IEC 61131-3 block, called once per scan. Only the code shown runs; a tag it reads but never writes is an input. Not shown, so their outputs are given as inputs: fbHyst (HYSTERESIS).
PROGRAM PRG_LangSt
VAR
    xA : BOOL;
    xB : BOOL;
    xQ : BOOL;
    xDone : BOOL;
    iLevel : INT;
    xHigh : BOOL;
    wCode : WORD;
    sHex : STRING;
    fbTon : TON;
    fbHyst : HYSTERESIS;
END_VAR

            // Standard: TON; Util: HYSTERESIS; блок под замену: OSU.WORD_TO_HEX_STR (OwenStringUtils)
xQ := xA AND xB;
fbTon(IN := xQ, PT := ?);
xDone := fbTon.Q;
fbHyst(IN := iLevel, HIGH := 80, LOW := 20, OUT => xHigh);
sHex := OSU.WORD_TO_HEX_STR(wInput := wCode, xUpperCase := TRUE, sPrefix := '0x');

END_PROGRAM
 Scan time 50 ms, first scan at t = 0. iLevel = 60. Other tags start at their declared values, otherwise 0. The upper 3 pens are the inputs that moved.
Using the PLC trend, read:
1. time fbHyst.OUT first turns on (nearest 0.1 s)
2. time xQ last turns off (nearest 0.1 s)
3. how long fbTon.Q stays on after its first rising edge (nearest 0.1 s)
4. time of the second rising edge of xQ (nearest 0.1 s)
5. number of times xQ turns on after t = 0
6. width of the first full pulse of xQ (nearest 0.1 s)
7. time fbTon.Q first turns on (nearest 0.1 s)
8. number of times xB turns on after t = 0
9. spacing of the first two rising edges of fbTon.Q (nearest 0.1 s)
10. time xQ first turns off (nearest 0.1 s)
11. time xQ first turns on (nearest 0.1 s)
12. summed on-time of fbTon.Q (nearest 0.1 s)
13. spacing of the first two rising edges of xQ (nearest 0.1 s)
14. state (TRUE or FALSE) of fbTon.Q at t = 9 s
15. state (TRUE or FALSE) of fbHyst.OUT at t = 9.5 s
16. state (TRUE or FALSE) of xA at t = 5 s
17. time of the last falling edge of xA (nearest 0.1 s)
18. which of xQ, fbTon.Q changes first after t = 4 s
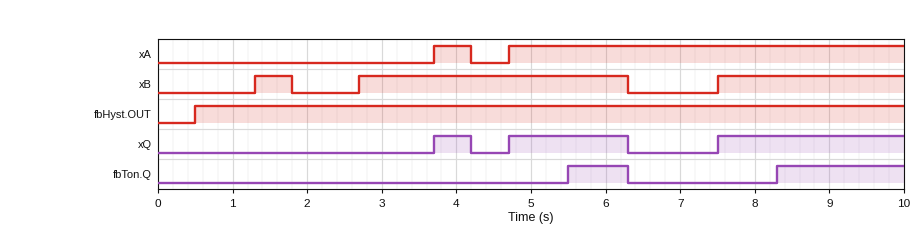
0.5 s
6.3 s
0.8 s
4.7 s
3
0.5 s
5.5 s
3
2.8 s
4.2 s
3.7 s
2.5 s
1.0 s
TRUE
TRUE
TRUE
4.2 s
xQ
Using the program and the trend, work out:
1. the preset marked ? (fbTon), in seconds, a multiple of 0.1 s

0.8 s
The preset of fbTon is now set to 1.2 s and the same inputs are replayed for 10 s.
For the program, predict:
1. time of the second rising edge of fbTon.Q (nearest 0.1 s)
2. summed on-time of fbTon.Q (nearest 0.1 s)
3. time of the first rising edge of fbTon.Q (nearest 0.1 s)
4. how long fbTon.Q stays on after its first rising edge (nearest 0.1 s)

8.7 s
1.7 s
5.9 s
0.4 s
